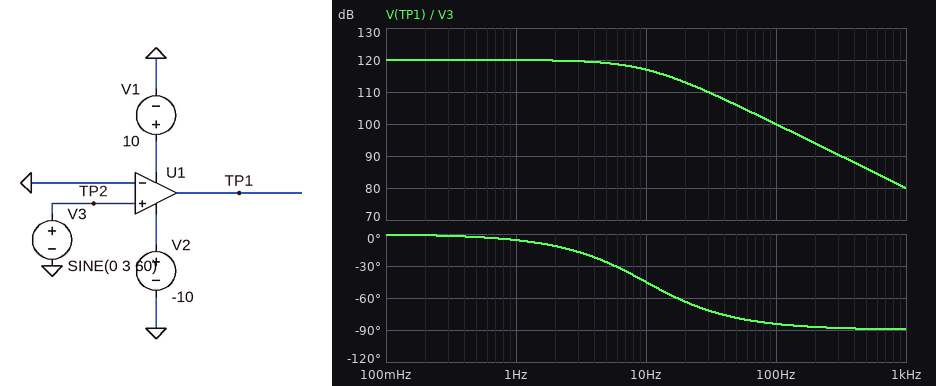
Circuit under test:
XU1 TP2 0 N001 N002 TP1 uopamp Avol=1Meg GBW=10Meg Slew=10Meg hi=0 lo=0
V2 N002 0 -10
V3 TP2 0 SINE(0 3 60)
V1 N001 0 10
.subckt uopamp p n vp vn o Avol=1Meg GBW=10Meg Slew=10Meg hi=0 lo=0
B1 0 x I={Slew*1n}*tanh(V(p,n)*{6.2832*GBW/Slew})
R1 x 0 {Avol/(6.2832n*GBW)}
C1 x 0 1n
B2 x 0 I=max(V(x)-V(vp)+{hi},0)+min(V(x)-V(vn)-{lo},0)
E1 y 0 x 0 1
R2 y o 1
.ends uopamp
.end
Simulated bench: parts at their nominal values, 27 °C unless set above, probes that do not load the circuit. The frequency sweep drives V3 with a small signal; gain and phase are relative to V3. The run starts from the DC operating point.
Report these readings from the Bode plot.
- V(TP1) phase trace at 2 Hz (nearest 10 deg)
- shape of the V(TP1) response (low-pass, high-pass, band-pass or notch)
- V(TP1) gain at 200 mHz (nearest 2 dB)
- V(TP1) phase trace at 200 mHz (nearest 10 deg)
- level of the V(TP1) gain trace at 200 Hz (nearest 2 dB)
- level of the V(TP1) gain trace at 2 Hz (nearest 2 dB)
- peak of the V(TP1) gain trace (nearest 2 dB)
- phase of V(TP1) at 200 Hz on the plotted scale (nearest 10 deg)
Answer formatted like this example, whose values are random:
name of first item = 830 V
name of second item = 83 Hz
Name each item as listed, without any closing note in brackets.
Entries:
V(TP1) phase trace at 2 Hz = -10 deg
shape of the V(TP1) response = low-pass
V(TP1) gain at 200 mHz = 120 dB
V(TP1) phase trace at 200 mHz = 0 deg
level of the V(TP1) gain trace at 200 Hz = 94 dB
level of the V(TP1) gain trace at 2 Hz = 120 dB
peak of the V(TP1) gain trace = 120 dB
phase of V(TP1) at 200 Hz on the plotted scale = -90 deg
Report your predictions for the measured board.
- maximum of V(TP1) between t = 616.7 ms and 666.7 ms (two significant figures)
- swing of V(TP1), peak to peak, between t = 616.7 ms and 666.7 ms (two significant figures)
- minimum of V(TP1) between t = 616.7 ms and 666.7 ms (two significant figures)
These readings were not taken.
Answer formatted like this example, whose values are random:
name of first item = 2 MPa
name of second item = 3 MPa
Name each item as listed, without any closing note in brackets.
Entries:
maximum of V(TP1) between t = 616.7 ms and 666.7 ms = 10 V
swing of V(TP1), peak to peak, between t = 616.7 ms and 666.7 ms = 20 V
minimum of V(TP1) between t = 616.7 ms and 666.7 ms = -10 V
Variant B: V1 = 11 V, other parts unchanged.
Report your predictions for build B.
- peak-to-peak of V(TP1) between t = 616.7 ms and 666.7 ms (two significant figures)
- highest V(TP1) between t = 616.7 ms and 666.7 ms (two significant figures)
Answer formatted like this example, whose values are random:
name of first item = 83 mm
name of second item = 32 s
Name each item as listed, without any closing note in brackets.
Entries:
peak-to-peak of V(TP1) between t = 616.7 ms and 666.7 ms = 21 V
highest V(TP1) between t = 616.7 ms and 666.7 ms = 11 V
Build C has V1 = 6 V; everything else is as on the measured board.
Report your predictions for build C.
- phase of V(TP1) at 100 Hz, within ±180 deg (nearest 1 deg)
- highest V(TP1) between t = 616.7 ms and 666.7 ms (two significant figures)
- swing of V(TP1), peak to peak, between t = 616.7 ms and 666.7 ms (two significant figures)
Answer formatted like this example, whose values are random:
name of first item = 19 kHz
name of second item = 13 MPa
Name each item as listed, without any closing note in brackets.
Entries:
phase of V(TP1) at 100 Hz, within ±180 deg = -84 deg
highest V(TP1) between t = 616.7 ms and 666.7 ms = 6.0 V
swing of V(TP1), peak to peak, between t = 616.7 ms and 666.7 ms = 16 V
